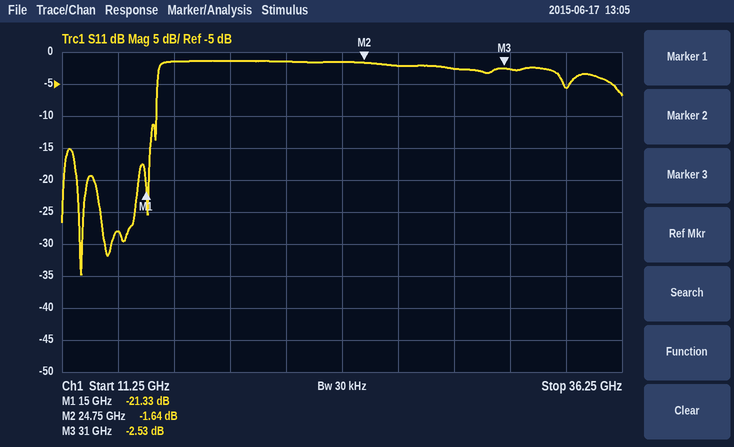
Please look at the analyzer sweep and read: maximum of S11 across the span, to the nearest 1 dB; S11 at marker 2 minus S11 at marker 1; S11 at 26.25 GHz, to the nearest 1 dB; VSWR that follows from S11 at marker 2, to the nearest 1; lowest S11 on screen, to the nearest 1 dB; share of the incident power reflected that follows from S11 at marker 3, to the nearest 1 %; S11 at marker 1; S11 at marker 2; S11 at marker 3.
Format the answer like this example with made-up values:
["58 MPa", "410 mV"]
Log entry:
["-1 dB", "19.69 dB", "-2 dB", "11", "-35 dB", "56 %", "-21.33 dB", "-1.64 dB", "-2.53 dB"]
